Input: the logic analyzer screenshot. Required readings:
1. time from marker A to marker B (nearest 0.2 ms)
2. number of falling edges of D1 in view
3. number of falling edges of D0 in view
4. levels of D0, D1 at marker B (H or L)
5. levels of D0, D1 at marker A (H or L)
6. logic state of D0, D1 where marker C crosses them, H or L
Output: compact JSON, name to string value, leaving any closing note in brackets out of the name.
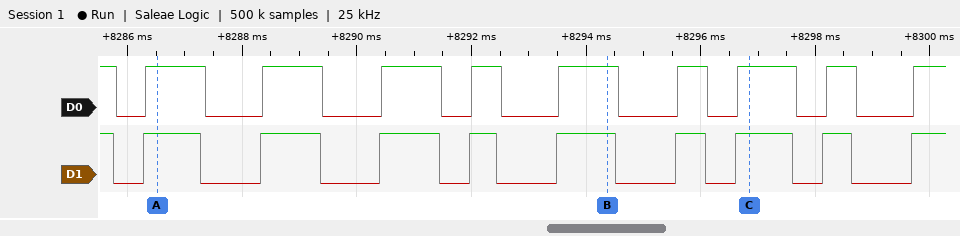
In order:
{"time from marker A to marker B": "7.8 ms", "number of falling edges of D1 in view": "9", "number of falling edges of D0 in view": "9", "levels of D0, D1 at marker B": "D0=H, D1=H", "levels of D0, D1 at marker A": "D0=H, D1=H", "logic state of D0, D1 where marker C crosses them, H or L": "D0=H, D1=H"}
